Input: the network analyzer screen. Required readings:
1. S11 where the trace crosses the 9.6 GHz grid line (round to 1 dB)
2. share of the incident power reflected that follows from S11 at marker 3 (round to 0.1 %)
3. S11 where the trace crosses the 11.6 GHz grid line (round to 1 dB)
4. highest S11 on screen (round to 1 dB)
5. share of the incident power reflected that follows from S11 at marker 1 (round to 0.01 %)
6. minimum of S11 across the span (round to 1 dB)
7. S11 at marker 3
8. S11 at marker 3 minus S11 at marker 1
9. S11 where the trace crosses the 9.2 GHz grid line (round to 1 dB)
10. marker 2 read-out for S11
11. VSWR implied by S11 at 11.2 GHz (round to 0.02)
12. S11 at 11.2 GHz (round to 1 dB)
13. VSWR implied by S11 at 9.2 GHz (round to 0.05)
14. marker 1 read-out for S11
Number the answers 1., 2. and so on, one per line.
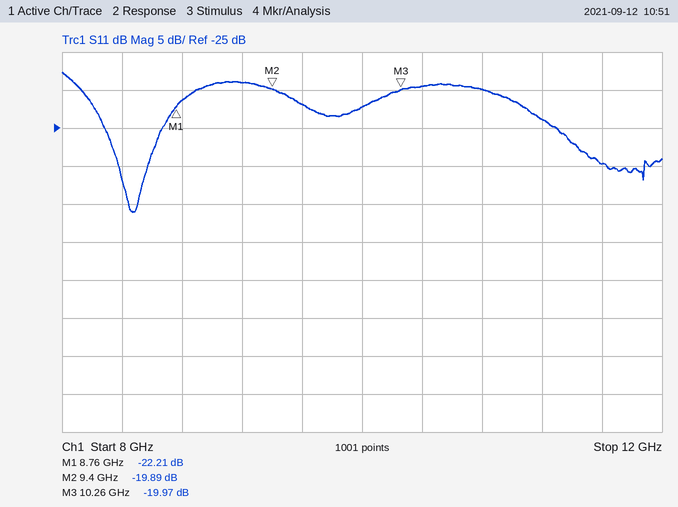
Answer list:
1. -22 dB
2. 1.0 %
3. -30 dB
4. -18 dB
5. 0.60 %
6. -36 dB
7. -19.97 dB
8. 2.24 dB
9. -19 dB
10. -19.89 dB
11. 1.14
12. -24 dB
13. 1.25
14. -22.21 dB
